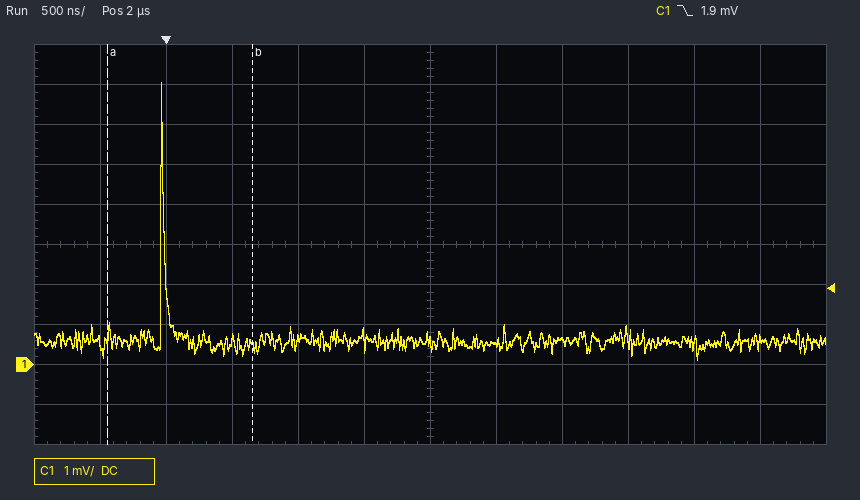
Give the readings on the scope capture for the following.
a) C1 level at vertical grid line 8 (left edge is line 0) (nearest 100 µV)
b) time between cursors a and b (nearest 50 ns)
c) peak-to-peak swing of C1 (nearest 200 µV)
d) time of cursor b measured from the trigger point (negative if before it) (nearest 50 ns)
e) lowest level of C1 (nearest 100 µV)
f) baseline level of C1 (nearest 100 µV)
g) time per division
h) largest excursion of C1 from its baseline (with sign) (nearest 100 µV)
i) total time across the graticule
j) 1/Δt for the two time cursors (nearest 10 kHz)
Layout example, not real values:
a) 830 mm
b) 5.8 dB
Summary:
a) 600 µV
b) 1.10 µs
c) 7.0 mV
d) +650 ns
e) 100 µV
f) 600 µV
g) 500 ns
h) +6.5 mV
i) 6 µs
j) 910 kHz
